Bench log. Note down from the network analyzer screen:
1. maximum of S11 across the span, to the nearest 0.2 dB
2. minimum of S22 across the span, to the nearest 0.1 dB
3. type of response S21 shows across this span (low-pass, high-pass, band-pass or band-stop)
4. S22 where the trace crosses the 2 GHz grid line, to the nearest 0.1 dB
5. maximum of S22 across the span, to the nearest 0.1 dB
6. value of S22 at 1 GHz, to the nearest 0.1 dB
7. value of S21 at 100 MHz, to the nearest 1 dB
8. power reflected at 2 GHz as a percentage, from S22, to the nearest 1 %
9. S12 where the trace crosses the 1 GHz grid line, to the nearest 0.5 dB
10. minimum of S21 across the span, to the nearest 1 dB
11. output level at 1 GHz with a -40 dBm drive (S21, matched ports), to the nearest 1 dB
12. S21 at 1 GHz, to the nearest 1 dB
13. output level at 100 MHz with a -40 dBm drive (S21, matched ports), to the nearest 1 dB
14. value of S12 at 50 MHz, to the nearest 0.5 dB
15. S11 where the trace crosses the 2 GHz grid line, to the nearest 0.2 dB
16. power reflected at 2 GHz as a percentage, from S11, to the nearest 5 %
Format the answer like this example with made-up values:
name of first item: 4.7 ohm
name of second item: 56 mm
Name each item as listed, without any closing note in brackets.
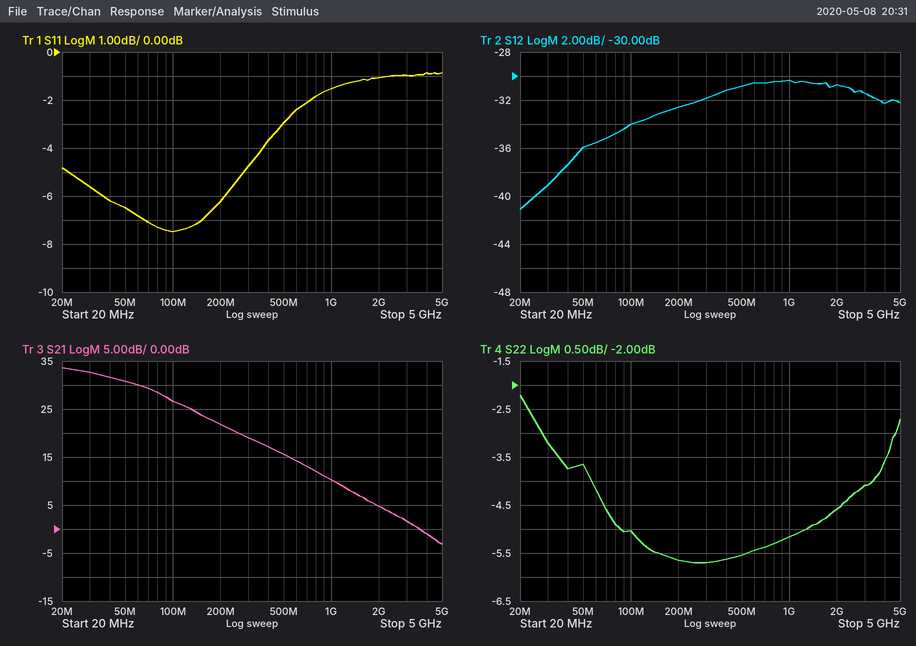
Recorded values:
maximum of S11 across the span, to the nearest 0.2 dB: -0.8 dB
minimum of S22 across the span, to the nearest 0.1 dB: -5.7 dB
type of response S21 shows across this span: low-pass
S22 where the trace crosses the 2 GHz grid line, to the nearest 0.1 dB: -4.6 dB
maximum of S22 across the span, to the nearest 0.1 dB: -2.2 dB
value of S22 at 1 GHz, to the nearest 0.1 dB: -5.2 dB
value of S21 at 100 MHz, to the nearest 1 dB: 27 dB
power reflected at 2 GHz as a percentage, from S22, to the nearest 1 %: 35 %
S12 where the trace crosses the 1 GHz grid line, to the nearest 0.5 dB: -30.5 dB
minimum of S21 across the span, to the nearest 1 dB: -3 dB
output level at 1 GHz with a -40 dBm drive (S21, matched ports), to the nearest 1 dB: -30 dBm
S21 at 1 GHz, to the nearest 1 dB: 10 dB
output level at 100 MHz with a -40 dBm drive (S21, matched ports), to the nearest 1 dB: -13 dBm
value of S12 at 50 MHz, to the nearest 0.5 dB: -36.0 dB
S11 where the trace crosses the 2 GHz grid line, to the nearest 0.2 dB: -1.0 dB
power reflected at 2 GHz as a percentage, from S11, to the nearest 5 %: 80 %
